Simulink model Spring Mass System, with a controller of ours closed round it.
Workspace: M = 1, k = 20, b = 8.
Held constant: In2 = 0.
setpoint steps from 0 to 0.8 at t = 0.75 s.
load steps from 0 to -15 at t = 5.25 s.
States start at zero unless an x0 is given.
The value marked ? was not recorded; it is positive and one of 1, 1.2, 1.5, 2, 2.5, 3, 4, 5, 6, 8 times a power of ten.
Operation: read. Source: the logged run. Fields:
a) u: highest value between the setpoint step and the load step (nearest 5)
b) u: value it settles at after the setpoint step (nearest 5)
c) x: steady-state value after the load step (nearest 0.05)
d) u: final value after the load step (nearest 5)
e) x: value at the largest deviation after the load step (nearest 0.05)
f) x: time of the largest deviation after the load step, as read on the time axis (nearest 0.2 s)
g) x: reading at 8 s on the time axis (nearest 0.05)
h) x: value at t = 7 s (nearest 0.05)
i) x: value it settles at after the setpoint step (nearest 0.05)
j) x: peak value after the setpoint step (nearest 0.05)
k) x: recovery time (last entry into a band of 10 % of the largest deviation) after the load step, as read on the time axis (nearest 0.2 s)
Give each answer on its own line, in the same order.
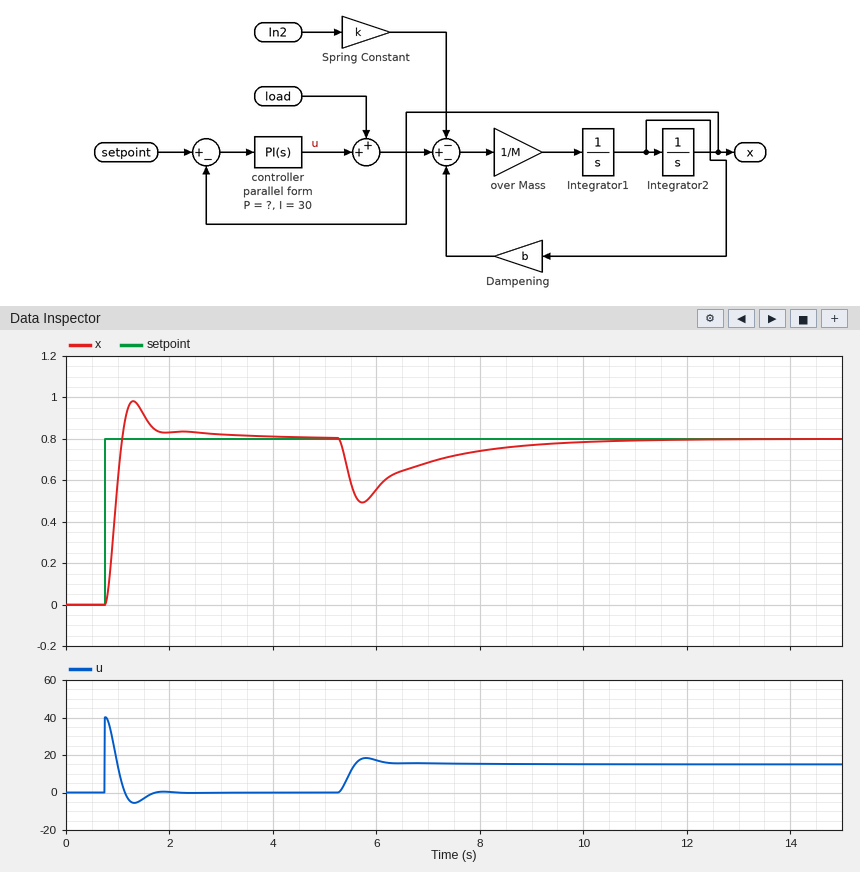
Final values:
40
0
0.80
15
0.50
5.8 s
0.75
0.70
0.80
1.00
9.0 s
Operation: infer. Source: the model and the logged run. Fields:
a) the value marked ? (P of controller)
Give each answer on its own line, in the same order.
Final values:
50
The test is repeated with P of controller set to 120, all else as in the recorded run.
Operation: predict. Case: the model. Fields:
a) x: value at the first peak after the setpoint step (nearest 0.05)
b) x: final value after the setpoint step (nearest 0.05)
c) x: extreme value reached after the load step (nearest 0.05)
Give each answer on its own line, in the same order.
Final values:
1.05
0.80
0.65
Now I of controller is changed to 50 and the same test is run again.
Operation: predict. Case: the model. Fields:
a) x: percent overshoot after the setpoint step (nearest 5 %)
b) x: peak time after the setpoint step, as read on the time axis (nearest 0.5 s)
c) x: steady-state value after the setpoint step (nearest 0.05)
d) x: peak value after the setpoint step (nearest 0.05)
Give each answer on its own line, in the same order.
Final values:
30 %
1.5 s
0.80
1.05
